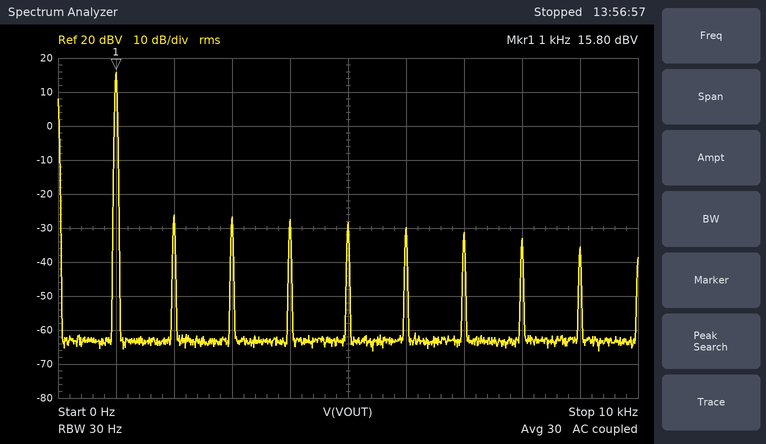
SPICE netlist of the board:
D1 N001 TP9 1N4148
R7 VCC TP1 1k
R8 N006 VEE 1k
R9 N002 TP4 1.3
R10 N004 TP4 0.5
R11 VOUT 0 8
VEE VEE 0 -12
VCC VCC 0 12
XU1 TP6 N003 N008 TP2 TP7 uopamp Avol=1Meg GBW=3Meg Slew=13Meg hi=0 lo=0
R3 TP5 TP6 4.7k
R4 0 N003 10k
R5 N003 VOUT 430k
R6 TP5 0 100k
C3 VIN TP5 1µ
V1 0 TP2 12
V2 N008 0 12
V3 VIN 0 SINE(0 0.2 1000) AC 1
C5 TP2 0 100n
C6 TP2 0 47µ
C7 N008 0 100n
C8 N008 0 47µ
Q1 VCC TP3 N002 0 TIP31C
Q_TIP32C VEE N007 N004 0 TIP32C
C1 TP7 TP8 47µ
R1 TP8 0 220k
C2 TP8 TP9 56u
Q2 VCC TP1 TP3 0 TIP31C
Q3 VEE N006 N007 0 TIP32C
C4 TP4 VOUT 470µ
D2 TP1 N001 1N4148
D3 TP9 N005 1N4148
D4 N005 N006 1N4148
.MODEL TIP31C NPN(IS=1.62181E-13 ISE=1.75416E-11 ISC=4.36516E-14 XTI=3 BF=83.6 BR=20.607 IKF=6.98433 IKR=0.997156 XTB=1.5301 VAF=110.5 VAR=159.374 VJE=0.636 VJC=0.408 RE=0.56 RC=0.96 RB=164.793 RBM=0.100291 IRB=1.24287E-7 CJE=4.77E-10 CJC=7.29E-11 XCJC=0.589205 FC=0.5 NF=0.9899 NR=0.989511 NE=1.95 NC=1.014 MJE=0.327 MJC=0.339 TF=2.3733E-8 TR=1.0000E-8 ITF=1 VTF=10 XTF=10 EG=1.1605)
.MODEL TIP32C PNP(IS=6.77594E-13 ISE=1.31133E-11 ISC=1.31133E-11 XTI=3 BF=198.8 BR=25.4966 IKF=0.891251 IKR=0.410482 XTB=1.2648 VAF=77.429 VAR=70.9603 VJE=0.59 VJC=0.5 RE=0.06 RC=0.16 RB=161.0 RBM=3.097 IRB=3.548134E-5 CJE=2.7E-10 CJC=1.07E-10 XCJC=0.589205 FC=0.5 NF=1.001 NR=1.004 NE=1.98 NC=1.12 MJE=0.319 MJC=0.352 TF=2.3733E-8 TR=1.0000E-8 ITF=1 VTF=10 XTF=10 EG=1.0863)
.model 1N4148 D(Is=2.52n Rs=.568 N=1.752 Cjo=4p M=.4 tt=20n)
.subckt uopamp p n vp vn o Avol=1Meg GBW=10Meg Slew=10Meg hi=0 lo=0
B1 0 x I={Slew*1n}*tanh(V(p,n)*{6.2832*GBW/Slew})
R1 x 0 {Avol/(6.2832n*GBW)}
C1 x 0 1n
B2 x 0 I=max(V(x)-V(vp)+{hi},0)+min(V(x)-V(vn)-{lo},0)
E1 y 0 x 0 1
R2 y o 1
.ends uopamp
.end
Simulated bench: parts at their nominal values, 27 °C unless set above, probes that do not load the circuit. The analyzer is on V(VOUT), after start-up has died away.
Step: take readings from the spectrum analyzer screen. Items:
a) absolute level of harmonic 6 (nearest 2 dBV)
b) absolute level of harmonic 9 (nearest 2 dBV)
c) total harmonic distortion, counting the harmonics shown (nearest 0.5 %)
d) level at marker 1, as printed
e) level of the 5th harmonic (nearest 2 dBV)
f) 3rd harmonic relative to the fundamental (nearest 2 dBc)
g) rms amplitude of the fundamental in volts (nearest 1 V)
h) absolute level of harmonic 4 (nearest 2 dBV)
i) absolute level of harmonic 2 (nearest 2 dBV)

-30 dBV
-36 dBV
1.5 %
15.80 dBV
-28 dBV
-42 dBc
6 V
-28 dBV
-26 dBV
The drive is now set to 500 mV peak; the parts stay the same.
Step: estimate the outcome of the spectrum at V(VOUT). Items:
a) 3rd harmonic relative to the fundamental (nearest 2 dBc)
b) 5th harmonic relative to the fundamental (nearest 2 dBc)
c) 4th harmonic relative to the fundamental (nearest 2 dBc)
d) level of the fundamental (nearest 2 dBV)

-12 dBc
-22 dBc
-58 dBc
18 dBV
